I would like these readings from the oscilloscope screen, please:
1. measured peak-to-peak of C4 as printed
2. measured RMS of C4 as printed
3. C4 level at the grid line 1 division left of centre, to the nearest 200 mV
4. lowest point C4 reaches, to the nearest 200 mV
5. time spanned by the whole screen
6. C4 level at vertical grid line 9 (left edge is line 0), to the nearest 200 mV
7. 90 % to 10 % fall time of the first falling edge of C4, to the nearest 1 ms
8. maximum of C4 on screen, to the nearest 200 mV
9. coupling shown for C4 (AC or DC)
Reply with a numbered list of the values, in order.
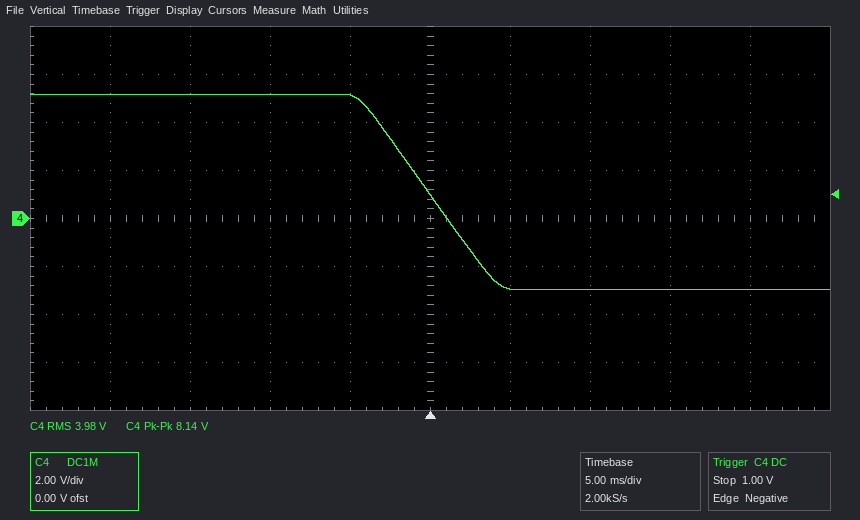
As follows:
1. 8.14 V
2. 3.98 V
3. 5.2 V
4. -3.0 V
5. 50 ms
6. -3.0 V
7. 7 ms
8. 5.2 V
9. DC
